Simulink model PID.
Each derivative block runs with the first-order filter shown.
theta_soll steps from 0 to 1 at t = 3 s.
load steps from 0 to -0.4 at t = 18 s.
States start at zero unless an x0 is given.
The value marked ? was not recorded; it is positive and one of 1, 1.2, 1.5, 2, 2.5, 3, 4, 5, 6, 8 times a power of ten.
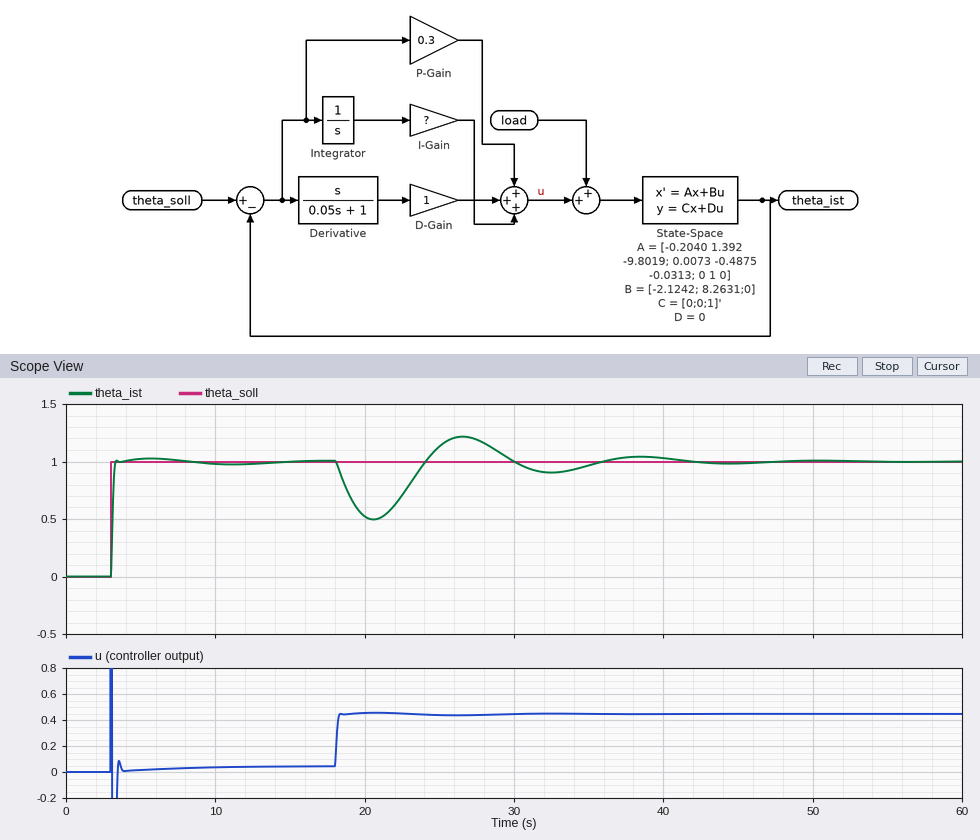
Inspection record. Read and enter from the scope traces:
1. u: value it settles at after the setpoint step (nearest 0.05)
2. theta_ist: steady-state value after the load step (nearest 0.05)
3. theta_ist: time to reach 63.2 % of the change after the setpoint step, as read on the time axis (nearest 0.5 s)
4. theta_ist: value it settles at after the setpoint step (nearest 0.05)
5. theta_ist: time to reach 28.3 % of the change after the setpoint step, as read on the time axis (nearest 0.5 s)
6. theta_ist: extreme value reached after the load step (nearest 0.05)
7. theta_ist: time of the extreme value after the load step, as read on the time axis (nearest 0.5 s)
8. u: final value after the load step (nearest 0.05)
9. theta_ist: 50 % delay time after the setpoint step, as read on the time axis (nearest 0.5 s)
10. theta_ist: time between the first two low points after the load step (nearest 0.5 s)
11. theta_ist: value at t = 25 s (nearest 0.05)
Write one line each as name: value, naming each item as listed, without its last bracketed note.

u: value it settles at after the setpoint step: 0.05
theta_ist: steady-state value after the load step: 1.00
theta_ist: time to reach 63.2 % of the change after the setpoint step, as read on the time axis: 3.0 s
theta_ist: value it settles at after the setpoint step: 1.00
theta_ist: time to reach 28.3 % of the change after the setpoint step, as read on the time axis: 3.0 s
theta_ist: extreme value reached after the load step: 0.50
theta_ist: time of the extreme value after the load step, as read on the time axis: 20.5 s
u: final value after the load step: 0.45
theta_ist: 50 % delay time after the setpoint step, as read on the time axis: 3.0 s
theta_ist: time between the first two low points after the load step: 12.0 s
theta_ist: value at t = 25 s: 1.15
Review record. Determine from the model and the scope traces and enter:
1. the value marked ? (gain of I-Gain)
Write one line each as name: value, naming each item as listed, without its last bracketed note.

the value marked ?: 0.3
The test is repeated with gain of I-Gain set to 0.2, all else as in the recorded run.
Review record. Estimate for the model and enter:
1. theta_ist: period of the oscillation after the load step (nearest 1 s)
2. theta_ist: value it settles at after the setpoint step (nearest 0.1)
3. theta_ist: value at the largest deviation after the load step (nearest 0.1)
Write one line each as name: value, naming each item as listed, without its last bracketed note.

theta_ist: period of the oscillation after the load step: 15 s
theta_ist: value it settles at after the setpoint step: 1.0
theta_ist: value at the largest deviation after the load step: 0.4
